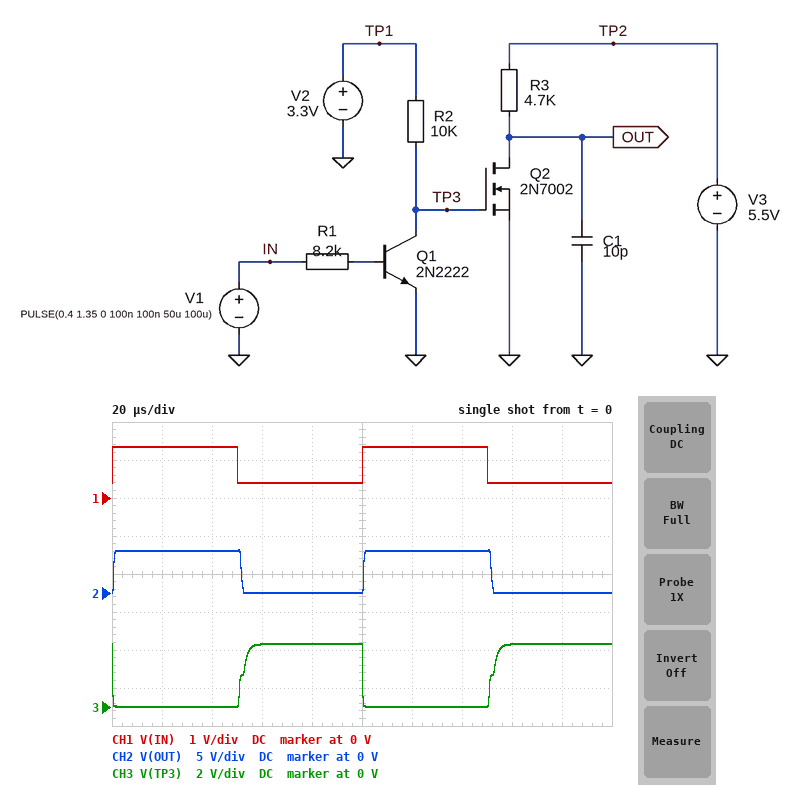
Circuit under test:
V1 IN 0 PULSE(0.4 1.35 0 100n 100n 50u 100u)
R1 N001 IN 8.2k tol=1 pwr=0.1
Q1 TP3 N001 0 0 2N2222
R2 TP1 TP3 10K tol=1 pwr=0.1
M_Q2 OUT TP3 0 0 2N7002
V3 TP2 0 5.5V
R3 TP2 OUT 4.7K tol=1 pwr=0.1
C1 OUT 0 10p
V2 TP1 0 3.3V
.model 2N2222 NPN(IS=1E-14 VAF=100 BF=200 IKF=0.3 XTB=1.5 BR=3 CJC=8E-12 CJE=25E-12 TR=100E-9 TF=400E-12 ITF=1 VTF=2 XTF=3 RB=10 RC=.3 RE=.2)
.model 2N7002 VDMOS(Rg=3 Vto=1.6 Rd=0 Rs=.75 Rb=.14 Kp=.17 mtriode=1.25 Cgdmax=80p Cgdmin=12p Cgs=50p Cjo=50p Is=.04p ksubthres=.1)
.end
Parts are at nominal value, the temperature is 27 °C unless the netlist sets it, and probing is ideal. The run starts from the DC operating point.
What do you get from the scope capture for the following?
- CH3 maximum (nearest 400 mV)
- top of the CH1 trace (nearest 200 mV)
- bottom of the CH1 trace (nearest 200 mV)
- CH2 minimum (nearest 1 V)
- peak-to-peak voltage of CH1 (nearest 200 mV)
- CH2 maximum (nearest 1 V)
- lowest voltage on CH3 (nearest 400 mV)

3.2 V
1.4 V
400 mV
0 V
1.0 V
6 V
0 V
